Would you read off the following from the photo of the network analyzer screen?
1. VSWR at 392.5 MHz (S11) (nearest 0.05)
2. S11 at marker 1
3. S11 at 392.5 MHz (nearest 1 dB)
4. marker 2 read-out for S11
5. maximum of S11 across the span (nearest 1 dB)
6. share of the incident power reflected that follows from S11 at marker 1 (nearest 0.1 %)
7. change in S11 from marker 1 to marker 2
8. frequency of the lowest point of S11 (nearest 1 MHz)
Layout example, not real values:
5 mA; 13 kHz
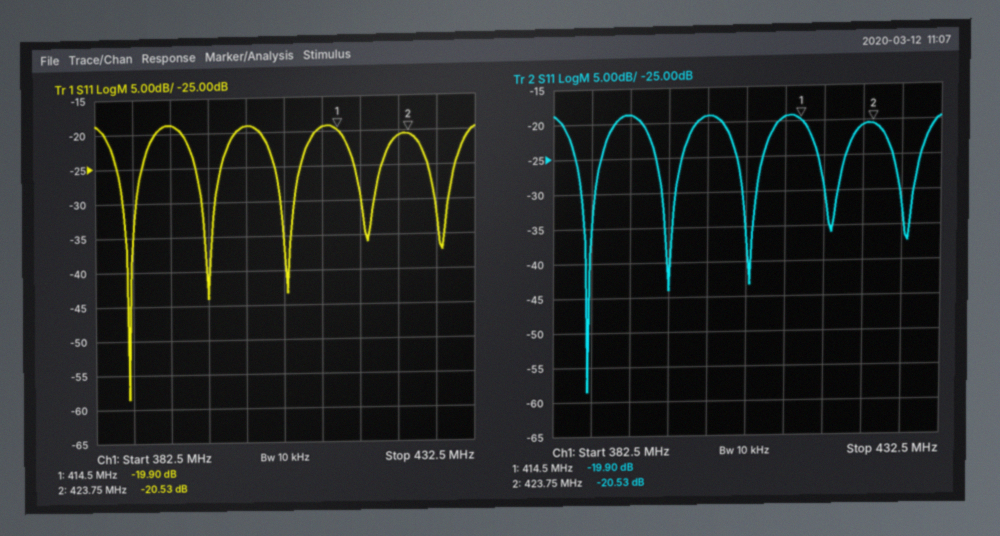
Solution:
1.25; -19.90 dB; -19 dB; -20.53 dB; -19 dB; 1.0 %; -0.63 dB; 387 MHz
